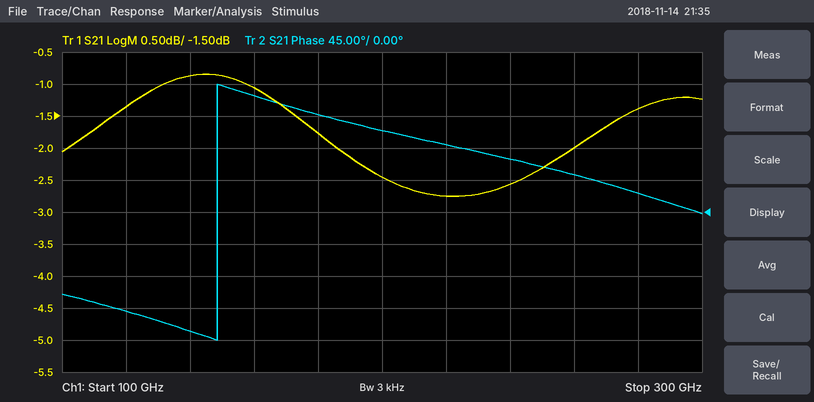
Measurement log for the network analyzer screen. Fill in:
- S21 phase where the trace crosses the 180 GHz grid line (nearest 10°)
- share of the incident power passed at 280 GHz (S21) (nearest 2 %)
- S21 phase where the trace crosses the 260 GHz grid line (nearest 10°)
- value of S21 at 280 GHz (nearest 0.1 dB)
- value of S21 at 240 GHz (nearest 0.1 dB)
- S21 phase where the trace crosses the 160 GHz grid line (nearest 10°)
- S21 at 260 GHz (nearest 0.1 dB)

140°
72 %
50°
-1.4 dB
-2.6 dB
160°
-2.0 dB
